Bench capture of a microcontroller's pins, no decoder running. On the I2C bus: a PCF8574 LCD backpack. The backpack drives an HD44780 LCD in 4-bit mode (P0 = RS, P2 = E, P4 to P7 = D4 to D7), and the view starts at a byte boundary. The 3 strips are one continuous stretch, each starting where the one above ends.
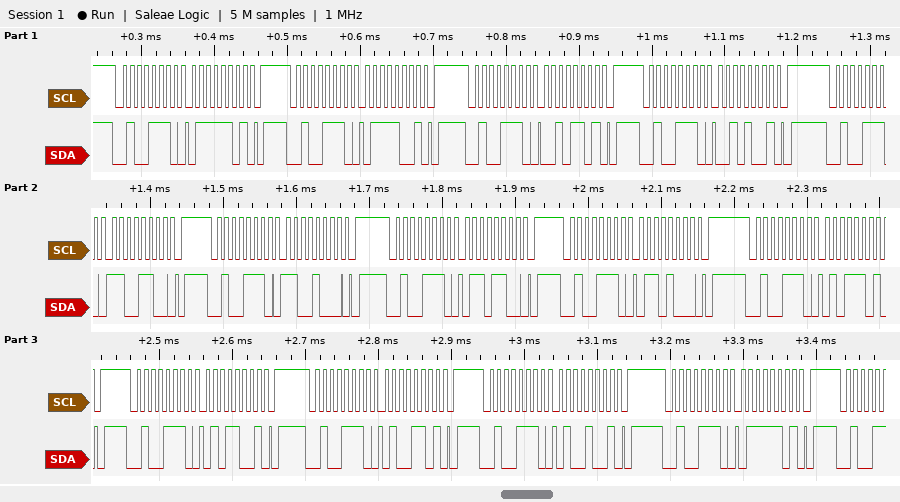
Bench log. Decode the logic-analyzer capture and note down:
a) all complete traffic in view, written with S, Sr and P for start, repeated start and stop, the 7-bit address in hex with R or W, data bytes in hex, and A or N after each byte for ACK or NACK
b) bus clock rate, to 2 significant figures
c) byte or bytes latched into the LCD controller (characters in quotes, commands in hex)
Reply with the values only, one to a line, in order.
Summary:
S 27W A 7D A P S 27W A 79 A P S 27W A 2D A P S 27W A 29 A P S 27W A CC A P S 27W A C8 A P S 27W A 6C A P S 27W A 68 A P S 27W A 5D A P S 27W A 59 A P S 27W A 4D A P S 27W A 49 A P S 27W A 7D A P
100 kHz
'r' 0xC6 'T'
